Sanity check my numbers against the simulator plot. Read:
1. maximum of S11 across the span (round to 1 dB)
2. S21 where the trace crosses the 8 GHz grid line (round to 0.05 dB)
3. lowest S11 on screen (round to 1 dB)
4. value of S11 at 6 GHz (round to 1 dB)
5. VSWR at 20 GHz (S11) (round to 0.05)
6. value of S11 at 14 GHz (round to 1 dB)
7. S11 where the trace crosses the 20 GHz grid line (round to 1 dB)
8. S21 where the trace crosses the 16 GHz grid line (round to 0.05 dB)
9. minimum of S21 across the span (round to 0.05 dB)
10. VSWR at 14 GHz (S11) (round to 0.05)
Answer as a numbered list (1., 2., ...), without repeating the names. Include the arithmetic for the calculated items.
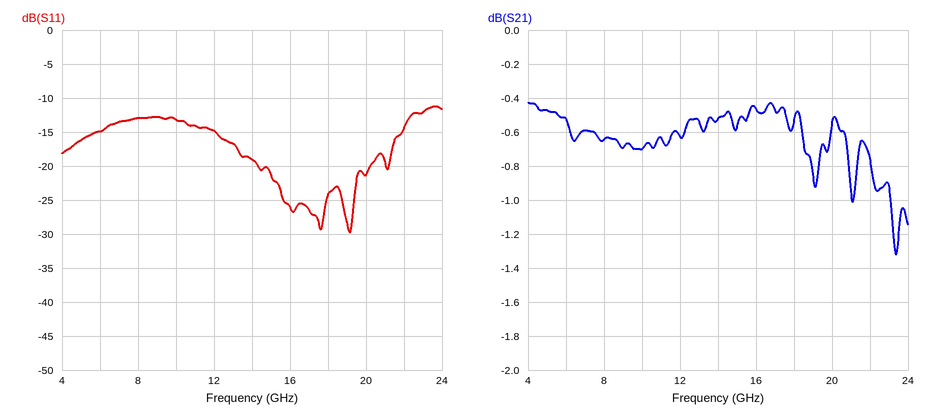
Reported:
1. -11 dB
2. -0.65 dB
3. -30 dB
4. -15 dB
5. |Γ| = 10^(-21/20) = 0.0891; VSWR = (1 + 0.0891)/(1 − 0.0891) ≈ 1.20
6. -19 dB
7. -21 dB
8. -0.45 dB
9. -1.30 dB
10. |Γ| = 10^(-19/20) = 0.1122; VSWR = (1 + 0.1122)/(1 − 0.1122) ≈ 1.25
